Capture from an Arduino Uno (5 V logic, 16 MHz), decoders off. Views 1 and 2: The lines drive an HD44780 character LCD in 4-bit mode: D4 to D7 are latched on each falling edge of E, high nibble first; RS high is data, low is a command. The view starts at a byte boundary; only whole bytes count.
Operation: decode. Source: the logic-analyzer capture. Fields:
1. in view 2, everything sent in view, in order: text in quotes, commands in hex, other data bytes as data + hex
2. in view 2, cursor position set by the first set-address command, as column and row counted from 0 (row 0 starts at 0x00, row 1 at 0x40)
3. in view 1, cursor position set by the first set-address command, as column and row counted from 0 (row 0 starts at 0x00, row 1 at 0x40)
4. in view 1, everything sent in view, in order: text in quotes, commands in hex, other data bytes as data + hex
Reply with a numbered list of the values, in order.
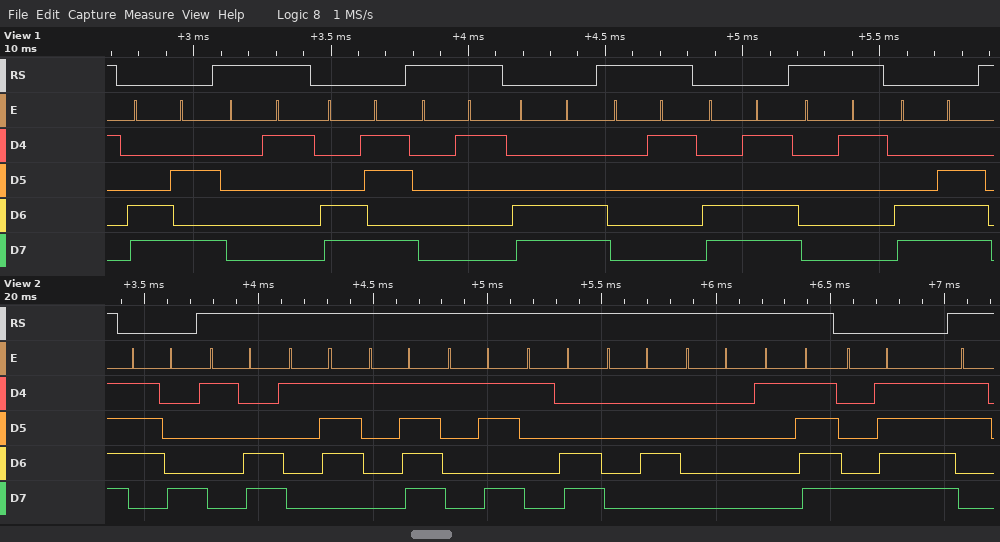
1. 0x78 data 1C 17 1F 1B 1C 04 00 1F 0x8F
2. column 15, row 0
3. column 10, row 1
4. 0xCA data 01 0xCB data 01 0xCC data 01 0xCD data 01 0xCE
